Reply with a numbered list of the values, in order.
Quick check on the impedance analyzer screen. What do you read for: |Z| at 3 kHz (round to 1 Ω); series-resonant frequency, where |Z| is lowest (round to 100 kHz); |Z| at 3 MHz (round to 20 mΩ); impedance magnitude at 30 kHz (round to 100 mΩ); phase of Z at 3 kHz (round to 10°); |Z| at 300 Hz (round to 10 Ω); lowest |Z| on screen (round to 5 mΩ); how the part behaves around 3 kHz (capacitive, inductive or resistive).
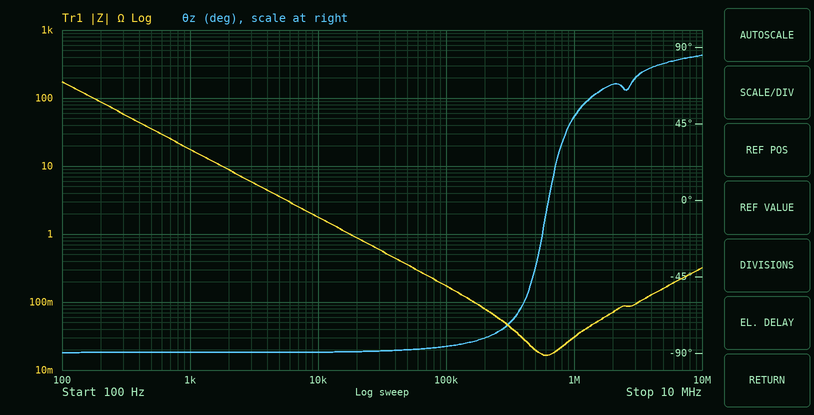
1. 6 Ω
2. 600 kHz
3. 100 mΩ
4. 600 mΩ
5. -90°
6. 60 Ω
7. 15 mΩ
8. capacitive
